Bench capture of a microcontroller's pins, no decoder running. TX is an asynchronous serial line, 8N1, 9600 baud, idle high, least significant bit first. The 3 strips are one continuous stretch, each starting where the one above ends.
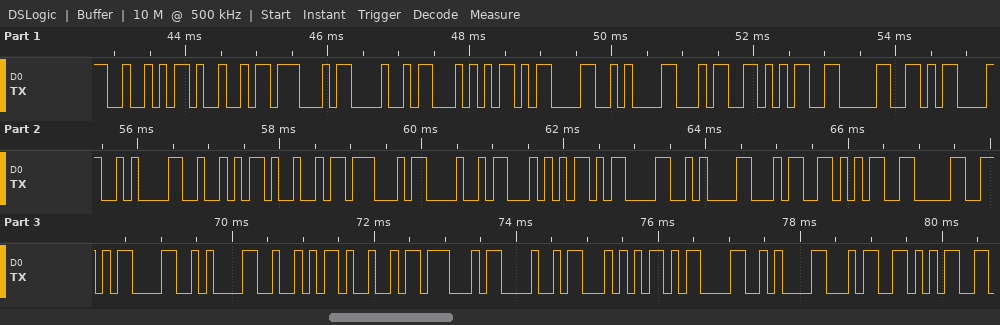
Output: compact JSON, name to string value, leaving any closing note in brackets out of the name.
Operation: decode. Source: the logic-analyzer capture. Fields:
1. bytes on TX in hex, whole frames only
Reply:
{"bytes on TX in hex, whole frames only": "52 49 47 48 54 0D 0A 34 35 30 0D 0A 52 49 47 48 54 0D 0A 34 35 30 0D 0A 52 49 47 48 54 0D 0A 34 35"}
